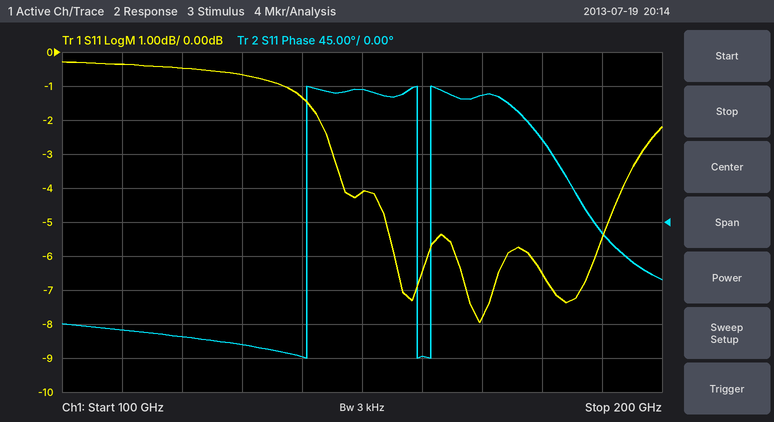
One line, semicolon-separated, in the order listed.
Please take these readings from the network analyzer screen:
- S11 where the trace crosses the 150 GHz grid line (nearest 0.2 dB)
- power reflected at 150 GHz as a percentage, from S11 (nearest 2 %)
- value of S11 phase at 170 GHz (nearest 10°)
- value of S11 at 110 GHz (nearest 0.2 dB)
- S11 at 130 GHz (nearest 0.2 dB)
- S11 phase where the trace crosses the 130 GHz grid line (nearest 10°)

-4.2 dB; 38 %; 170°; -0.4 dB; -0.6 dB; -160°
